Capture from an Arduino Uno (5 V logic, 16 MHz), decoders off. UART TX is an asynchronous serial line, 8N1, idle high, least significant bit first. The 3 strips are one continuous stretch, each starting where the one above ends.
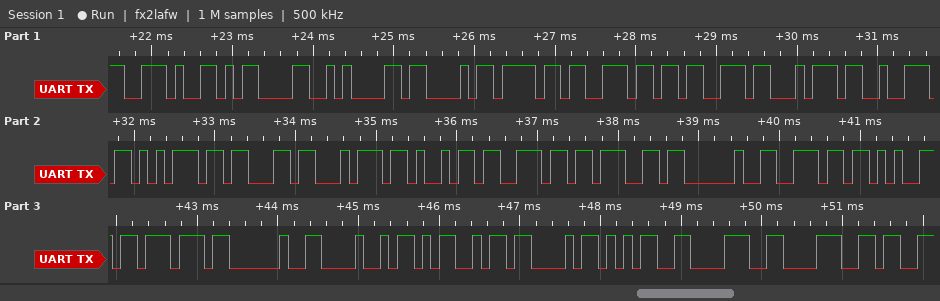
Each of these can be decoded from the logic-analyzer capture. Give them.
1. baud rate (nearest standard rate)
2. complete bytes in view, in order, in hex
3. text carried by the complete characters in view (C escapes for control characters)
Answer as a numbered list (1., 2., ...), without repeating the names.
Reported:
1. 9600 baud
2. 2E 0D 0A 43 6F 6E 73 74 72 75 63 74 69 6E 67 20 6E 65 77 20 48 4D 43 35 38 38
3. ".\r\nConstructing new HMC588"
